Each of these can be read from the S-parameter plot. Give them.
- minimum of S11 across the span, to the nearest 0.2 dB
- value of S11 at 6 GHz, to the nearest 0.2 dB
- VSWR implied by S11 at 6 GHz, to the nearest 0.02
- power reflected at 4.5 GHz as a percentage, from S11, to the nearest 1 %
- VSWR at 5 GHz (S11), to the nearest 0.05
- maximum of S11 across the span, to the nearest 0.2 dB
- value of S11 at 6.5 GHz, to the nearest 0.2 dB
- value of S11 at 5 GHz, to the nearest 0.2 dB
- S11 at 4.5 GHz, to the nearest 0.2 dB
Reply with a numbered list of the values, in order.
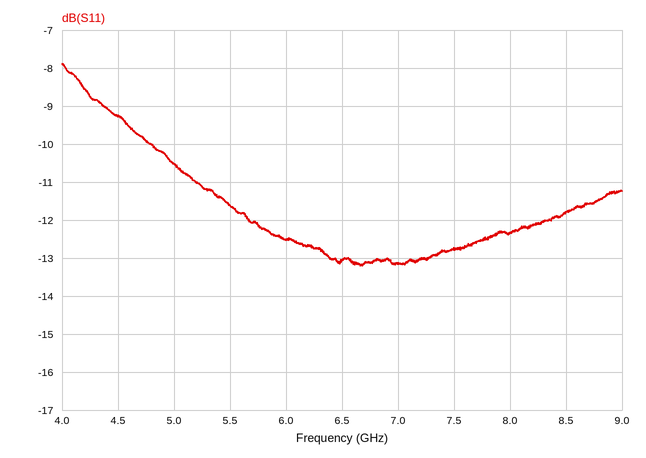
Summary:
1. -13.2 dB
2. -12.6 dB
3. 1.62
4. 12 %
5. 1.85
6. -7.8 dB
7. -13.0 dB
8. -10.6 dB
9. -9.2 dB
